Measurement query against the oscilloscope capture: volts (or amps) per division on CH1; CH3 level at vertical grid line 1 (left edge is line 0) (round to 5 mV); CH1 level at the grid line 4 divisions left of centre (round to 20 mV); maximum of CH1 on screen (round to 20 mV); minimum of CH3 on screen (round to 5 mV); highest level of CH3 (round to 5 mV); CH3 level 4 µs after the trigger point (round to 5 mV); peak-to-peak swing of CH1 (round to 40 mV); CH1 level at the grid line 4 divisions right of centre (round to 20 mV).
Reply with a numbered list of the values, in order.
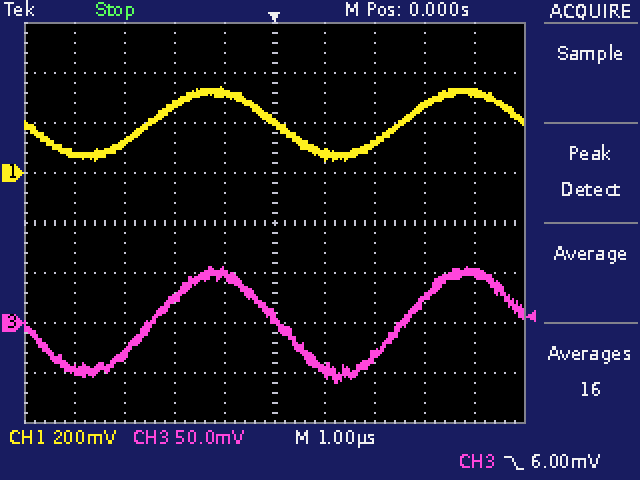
1. 200 mV
2. -45 mV
3. 80 mV
4. 340 mV
5. -60 mV
6. 55 mV
7. 50 mV
8. 280 mV
9. 320 mV
